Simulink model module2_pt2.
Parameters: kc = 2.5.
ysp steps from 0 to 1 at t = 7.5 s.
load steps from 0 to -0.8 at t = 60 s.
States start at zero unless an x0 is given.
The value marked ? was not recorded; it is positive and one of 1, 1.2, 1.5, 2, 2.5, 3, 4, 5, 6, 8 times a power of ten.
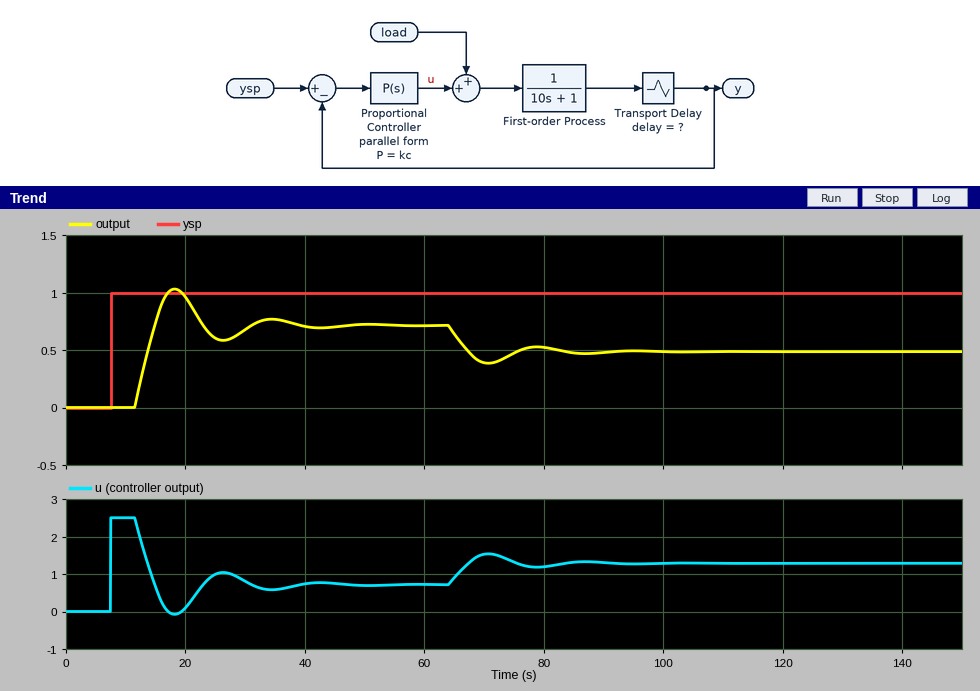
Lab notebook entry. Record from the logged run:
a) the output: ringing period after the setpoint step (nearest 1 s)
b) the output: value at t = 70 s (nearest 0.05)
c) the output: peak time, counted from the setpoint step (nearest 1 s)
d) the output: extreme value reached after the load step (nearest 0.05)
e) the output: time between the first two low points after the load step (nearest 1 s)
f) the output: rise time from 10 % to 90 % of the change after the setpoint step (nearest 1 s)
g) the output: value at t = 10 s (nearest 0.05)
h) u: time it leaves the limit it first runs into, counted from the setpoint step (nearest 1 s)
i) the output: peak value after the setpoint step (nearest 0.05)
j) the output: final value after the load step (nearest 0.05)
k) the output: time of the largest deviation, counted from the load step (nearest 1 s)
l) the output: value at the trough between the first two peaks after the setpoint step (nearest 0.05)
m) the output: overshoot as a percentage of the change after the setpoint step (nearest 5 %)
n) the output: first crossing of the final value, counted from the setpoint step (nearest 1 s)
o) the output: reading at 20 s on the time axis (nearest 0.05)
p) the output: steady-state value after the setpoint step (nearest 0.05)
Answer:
16 s
0.40
11 s
0.40
16 s
3 s
0.00
4 s
1.05
0.50
11 s
0.60
45 %
7 s
0.95
0.70
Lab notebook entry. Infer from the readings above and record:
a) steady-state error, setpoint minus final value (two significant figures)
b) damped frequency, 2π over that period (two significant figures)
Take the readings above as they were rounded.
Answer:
0.30
0.39 rad/s
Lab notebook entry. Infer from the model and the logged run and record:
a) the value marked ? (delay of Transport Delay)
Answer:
4
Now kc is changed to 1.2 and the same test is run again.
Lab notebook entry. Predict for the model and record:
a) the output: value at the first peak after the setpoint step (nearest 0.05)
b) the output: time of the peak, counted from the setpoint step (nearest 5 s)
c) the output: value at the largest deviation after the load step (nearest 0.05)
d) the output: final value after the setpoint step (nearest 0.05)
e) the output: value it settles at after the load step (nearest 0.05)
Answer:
0.60
15 s
0.15
0.55
0.20
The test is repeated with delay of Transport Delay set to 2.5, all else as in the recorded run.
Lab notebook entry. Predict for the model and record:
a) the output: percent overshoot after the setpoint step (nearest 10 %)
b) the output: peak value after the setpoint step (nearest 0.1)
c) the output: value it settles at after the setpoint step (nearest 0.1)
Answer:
20 %
0.8
0.7
